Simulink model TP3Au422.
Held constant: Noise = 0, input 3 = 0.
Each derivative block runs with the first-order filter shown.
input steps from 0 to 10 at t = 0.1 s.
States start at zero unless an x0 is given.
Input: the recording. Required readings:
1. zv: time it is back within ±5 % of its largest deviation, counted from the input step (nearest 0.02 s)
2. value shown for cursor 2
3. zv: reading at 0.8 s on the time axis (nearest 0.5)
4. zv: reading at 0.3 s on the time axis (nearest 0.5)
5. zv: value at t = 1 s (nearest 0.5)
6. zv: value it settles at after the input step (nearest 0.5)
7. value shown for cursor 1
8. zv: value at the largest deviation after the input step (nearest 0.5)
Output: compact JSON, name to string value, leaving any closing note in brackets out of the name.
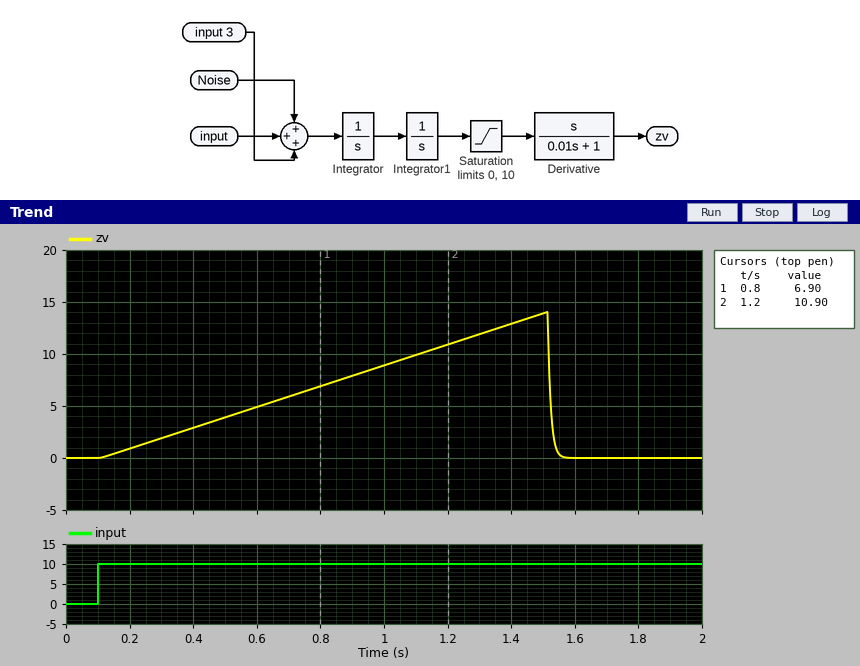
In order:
{"zv: time it is back within ±5 % of its largest deviation, counted from the input step": "1.44 s", "value shown for cursor 2": "10.90", "zv: reading at 0.8 s on the time axis": "7.0", "zv: reading at 0.3 s on the time axis": "2.0", "zv: value at t = 1 s": "9.0", "zv: value it settles at after the input step": "0.0", "value shown for cursor 1": "6.90", "zv: value at the largest deviation after the input step": "14.0"}
